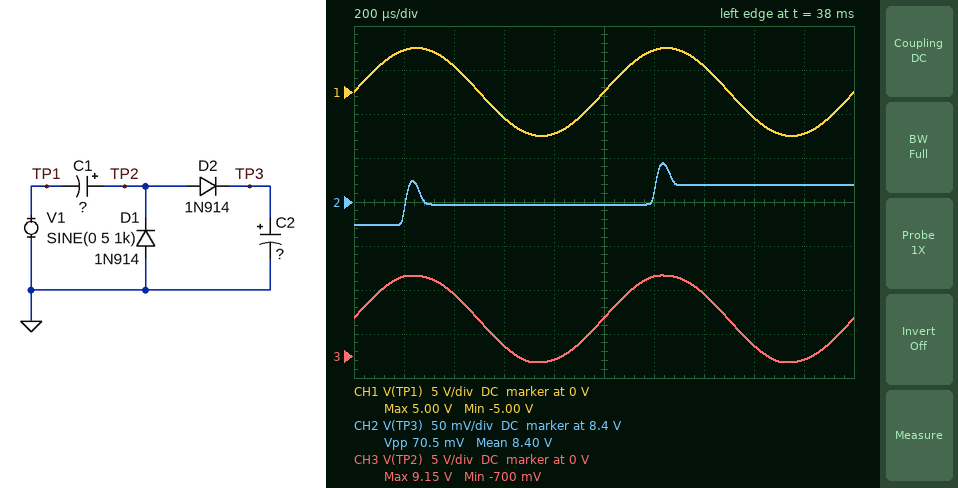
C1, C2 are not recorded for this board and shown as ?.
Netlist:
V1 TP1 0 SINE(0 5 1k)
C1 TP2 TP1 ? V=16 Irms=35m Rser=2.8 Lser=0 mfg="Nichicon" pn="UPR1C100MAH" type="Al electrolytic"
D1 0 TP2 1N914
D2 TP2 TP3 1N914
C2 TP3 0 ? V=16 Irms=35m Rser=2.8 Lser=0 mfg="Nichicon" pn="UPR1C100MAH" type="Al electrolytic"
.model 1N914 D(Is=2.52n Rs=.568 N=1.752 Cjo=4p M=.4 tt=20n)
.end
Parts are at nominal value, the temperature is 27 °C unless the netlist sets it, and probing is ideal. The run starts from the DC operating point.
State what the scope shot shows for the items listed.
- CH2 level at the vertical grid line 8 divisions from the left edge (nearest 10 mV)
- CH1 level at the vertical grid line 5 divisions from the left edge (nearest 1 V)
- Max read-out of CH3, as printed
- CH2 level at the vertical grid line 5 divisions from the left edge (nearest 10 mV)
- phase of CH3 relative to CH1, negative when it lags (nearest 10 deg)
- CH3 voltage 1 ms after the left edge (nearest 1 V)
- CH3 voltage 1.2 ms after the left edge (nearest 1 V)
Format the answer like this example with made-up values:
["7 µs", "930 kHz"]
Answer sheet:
["8.42 V", "0 V", "9.15 V", "8.40 V", "0 deg", "4 V", "9 V"]
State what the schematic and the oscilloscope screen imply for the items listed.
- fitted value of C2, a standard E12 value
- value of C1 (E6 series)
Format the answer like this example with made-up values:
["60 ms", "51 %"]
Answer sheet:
["33 µF", "3.3 µF"]
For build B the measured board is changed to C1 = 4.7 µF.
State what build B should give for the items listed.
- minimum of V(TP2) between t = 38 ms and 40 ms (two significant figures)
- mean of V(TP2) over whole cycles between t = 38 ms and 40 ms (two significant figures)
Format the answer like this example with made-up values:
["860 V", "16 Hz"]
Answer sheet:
["-690 mV", "4.3 V"]
